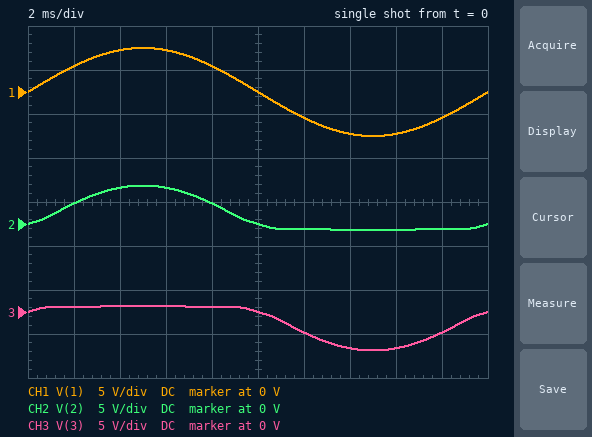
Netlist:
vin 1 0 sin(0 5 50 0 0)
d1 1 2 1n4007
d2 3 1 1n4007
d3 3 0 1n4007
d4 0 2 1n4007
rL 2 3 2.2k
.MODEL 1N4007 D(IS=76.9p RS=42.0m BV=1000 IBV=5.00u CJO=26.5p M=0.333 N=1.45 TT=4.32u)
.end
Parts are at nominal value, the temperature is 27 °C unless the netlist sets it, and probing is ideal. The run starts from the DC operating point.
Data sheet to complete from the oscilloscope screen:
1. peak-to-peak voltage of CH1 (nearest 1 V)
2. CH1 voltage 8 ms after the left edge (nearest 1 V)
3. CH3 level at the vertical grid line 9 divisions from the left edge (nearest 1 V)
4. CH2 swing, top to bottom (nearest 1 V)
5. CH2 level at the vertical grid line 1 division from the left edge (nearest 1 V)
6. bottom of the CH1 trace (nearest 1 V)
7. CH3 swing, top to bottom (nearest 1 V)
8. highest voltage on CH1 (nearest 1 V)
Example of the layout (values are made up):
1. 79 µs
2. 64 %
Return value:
1. 10 V
2. 3 V
3. -2 V
4. 5 V
5. 2 V
6. -5 V
7. 5 V
8. 5 V
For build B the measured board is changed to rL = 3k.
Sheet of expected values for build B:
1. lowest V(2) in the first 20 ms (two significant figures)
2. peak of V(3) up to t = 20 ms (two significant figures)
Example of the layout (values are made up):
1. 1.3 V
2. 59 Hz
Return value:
1. -620 mV
2. 620 mV
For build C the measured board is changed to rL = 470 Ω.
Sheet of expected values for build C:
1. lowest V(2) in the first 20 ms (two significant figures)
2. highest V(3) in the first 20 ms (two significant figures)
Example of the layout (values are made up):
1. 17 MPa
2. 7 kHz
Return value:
1. -690 mV
2. 690 mV
